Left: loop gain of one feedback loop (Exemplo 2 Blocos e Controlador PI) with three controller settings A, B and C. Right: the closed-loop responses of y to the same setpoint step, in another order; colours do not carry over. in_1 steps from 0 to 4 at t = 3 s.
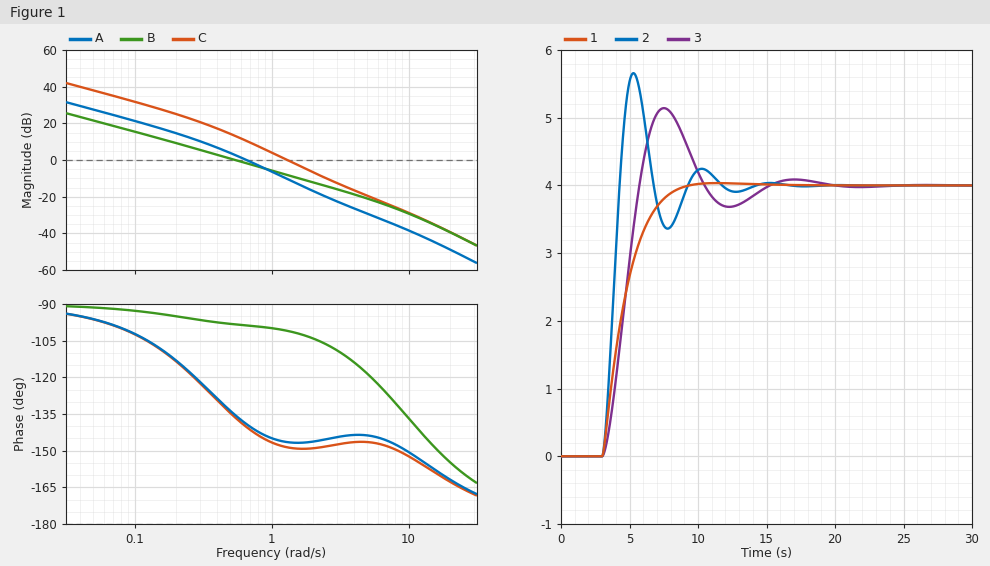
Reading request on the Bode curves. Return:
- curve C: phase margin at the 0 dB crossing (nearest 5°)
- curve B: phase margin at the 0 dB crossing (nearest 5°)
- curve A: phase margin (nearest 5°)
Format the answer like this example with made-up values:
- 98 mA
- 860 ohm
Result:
- 30°
- 80°
- 40°
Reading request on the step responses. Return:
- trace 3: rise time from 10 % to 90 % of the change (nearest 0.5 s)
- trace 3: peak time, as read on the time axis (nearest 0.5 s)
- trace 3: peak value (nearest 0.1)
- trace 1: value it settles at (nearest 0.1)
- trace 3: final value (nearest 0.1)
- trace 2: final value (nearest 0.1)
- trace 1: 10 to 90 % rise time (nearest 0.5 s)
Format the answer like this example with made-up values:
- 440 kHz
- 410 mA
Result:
- 2.0 s
- 7.5 s
- 5.1
- 4.0
- 4.0
- 4.0
- 3.5 s
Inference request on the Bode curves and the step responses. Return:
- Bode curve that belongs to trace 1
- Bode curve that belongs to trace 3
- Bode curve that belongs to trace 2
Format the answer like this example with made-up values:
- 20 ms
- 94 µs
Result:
- B
- A
- C
